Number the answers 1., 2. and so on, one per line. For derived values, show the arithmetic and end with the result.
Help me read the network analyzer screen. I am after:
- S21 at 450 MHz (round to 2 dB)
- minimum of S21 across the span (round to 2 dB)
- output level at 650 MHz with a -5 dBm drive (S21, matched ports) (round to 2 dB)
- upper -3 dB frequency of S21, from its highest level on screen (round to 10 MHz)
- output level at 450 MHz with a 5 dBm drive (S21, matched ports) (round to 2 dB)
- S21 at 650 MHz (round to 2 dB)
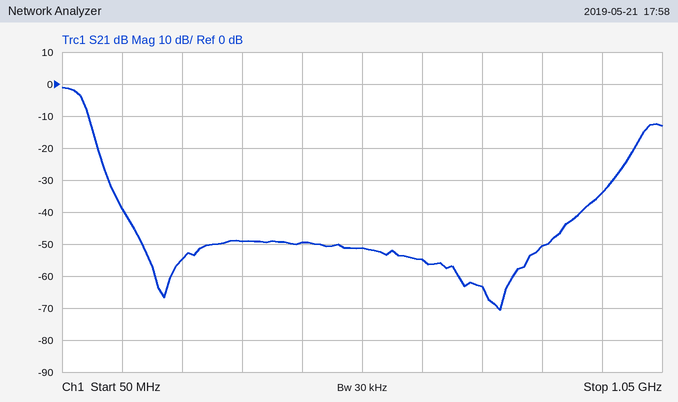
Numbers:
1. -50 dB
2. -70 dB
3. -5 dBm + (-54 dB) = -60 dBm
4. 80 MHz
5. 5 dBm + (-50 dB) = -44 dBm
6. -54 dB
